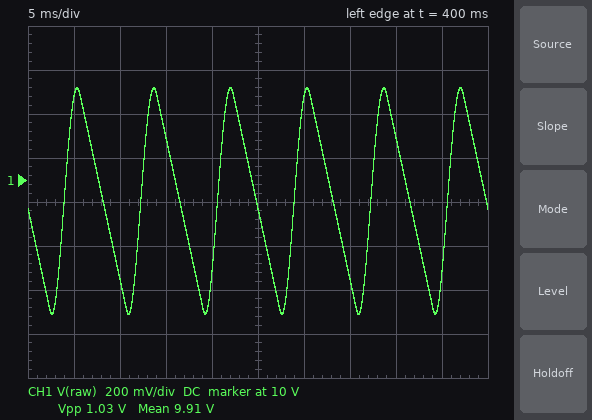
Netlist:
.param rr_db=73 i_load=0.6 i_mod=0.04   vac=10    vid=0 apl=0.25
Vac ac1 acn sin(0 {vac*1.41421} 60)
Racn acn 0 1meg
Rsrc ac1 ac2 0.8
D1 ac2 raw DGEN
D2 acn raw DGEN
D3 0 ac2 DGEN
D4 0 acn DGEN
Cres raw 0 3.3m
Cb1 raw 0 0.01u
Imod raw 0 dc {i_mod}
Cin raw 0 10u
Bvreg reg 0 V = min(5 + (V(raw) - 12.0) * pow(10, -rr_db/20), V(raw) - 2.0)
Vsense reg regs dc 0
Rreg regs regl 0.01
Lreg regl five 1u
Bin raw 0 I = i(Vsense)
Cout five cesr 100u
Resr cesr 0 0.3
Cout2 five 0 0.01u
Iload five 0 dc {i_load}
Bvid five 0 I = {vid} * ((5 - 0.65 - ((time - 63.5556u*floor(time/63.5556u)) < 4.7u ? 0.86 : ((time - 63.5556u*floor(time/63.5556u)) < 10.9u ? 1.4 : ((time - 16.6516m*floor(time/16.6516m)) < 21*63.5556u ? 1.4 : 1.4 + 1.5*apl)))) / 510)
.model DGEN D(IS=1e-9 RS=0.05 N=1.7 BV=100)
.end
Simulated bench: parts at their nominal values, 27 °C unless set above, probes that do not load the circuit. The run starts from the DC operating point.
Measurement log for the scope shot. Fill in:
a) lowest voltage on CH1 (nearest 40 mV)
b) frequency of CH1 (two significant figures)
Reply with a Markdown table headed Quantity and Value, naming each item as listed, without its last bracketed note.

| Quantity | Value |
|---|---|
| lowest voltage on CH1 | 9.40 V |
| frequency of CH1 | 120 Hz |
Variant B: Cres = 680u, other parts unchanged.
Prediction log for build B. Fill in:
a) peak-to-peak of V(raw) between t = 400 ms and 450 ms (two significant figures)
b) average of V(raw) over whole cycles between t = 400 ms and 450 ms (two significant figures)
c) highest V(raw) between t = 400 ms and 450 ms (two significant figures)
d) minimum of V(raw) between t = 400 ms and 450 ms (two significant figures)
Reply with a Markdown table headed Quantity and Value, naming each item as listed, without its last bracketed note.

| Quantity | Value |
|---|---|
| peak-to-peak of V(raw) between t = 400 ms and 450 ms | 4.6 V |
| average of V(raw) over whole cycles between t = 400 ms and 450 ms | 9.2 V |
| highest V(raw) between t = 400 ms and 450 ms | 11 V |
| minimum of V(raw) between t = 400 ms and 450 ms | 6.8 V |
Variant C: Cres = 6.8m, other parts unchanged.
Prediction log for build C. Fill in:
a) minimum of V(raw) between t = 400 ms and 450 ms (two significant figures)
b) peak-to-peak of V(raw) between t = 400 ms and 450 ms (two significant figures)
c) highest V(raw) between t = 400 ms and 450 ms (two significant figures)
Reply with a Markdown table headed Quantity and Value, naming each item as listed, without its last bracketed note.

| Quantity | Value |
|---|---|
| minimum of V(raw) between t = 400 ms and 450 ms | 9.7 V |
| peak-to-peak of V(raw) between t = 400 ms and 450 ms | 500 mV |
| highest V(raw) between t = 400 ms and 450 ms | 10 V |
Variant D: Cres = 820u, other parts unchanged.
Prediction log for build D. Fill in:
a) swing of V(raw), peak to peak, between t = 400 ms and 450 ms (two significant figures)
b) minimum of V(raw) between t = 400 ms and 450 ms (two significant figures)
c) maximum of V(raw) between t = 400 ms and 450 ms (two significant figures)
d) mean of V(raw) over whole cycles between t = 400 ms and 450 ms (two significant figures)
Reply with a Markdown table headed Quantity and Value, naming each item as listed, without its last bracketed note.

| Quantity | Value |
|---|---|
| swing of V(raw), peak to peak, between t = 400 ms and 450 ms | 3.9 V |
| minimum of V(raw) between t = 400 ms and 450 ms | 7.3 V |
| maximum of V(raw) between t = 400 ms and 450 ms | 11 V |
| mean of V(raw) over whole cycles between t = 400 ms and 450 ms | 9.4 V |
